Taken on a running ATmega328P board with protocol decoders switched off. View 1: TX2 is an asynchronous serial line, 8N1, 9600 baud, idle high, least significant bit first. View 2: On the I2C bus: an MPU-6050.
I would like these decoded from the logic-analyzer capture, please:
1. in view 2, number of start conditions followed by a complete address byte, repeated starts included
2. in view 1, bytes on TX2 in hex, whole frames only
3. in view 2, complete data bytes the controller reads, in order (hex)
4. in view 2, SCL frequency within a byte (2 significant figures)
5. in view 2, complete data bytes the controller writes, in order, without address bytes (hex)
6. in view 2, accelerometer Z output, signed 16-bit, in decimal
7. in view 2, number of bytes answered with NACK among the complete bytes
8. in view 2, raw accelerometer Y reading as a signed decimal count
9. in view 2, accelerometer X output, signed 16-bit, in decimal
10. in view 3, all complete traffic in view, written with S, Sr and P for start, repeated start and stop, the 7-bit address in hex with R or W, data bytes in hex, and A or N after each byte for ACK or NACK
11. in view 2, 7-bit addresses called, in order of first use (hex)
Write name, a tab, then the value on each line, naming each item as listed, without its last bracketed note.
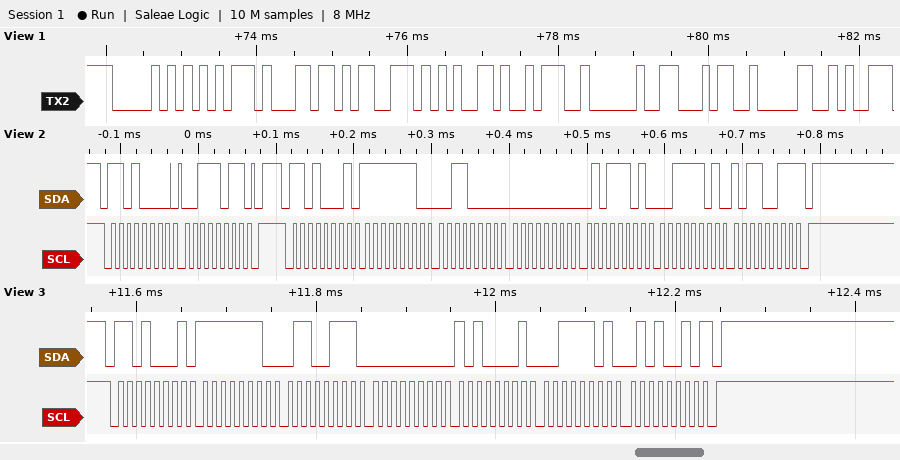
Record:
in view 2, number of start conditions followed by a complete address byte, repeated starts included	2
in view 1, bytes on TX2 in hex, whole frames only	50 75 6C 73 65 3A 20 34 30
in view 2, complete data bytes the controller reads, in order	FE 30 00 5D 3D B3
in view 2, SCL frequency within a byte	100 kHz
in view 2, complete data bytes the controller writes, in order, without address bytes	3B
in view 2, accelerometer Z output, signed 16-bit, in decimal	15795
in view 2, number of bytes answered with NACK among the complete bytes	1
in view 2, raw accelerometer Y reading as a signed decimal count	93
in view 2, accelerometer X output, signed 16-bit, in decimal	-464
in view 3, all complete traffic in view, written with S, Sr and P for start, repeated start and stop, the 7-bit address in hex with R or W, data bytes in hex, and A or N after each byte for ACK or NACK	S 68R A FE A 67 A 00 A A1 A 3D A 52 N P
in view 2, 7-bit addresses called, in order of first use	0x68
